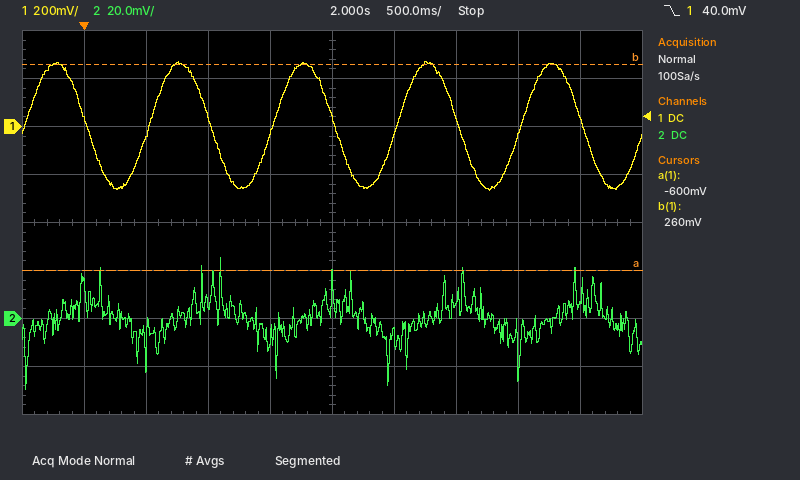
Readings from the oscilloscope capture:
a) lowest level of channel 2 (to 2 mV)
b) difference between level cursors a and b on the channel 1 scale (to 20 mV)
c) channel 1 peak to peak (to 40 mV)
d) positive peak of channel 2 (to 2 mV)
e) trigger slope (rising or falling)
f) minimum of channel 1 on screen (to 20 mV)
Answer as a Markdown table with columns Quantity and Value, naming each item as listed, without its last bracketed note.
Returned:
| Quantity | Value |
|---|---|
| lowest level of channel 2 | -30 mV |
| difference between level cursors a and b on the channel 1 scale | 860 mV |
| channel 1 peak to peak | 520 mV |
| positive peak of channel 2 | 26 mV |
| trigger slope | falling |
| minimum of channel 1 on screen | -260 mV |
